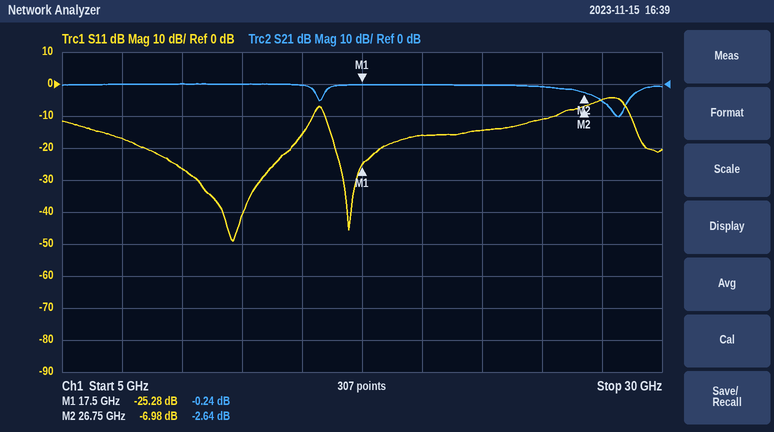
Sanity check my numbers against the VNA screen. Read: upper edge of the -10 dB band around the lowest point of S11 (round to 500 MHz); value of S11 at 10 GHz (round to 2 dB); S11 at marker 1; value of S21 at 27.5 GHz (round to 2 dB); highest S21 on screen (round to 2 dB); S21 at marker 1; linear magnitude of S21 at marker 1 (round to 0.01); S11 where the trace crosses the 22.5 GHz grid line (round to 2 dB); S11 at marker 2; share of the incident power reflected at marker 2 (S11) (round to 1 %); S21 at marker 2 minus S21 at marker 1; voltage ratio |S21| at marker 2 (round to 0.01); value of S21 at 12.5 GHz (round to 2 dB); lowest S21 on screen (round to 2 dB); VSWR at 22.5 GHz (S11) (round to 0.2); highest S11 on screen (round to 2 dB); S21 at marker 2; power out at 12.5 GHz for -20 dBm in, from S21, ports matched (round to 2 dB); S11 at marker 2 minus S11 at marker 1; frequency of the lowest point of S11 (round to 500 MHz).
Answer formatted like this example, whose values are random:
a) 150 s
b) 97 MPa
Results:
a) 15.5 GHz
b) -26 dB
c) -25.28 dB
d) -6 dB
e) 0 dB
f) -0.24 dB
g) 0.97
h) -14 dB
i) -6.98 dB
j) 20 %
k) -2.40 dB
l) 0.74
m) 0 dB
n) -10 dB
o) 1.4
p) -4 dB
q) -2.64 dB
r) -20 dBm
s) 18.30 dB
t) 12.0 GHz
